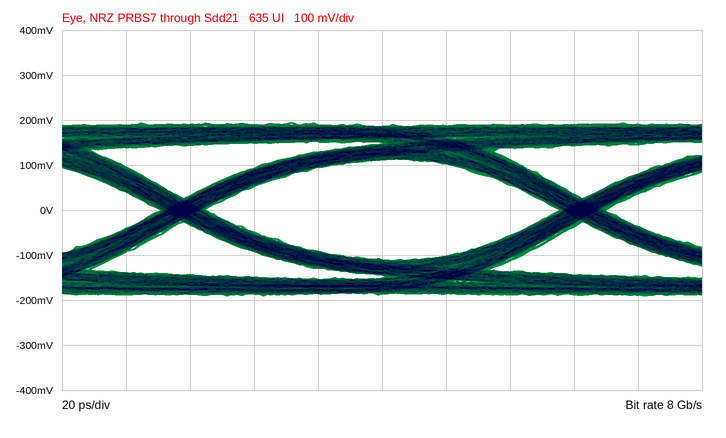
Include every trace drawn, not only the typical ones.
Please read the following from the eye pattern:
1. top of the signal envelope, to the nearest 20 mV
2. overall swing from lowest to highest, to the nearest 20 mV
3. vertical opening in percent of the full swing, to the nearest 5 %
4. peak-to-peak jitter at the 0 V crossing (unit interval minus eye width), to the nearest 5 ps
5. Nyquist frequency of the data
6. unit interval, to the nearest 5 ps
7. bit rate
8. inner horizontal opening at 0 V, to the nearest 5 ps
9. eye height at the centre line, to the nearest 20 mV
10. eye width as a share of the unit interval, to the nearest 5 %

200 mV
380 mV
60 %
15 ps
4 GHz
125 ps
8 Gb/s
110 ps
220 mV
90 %
